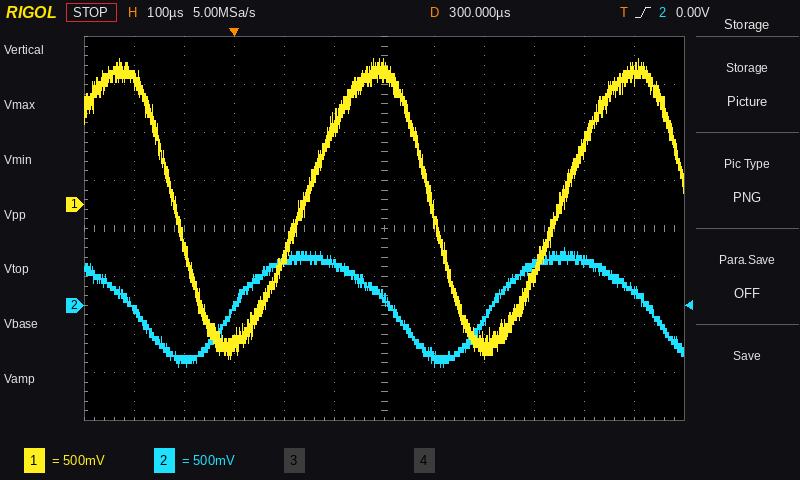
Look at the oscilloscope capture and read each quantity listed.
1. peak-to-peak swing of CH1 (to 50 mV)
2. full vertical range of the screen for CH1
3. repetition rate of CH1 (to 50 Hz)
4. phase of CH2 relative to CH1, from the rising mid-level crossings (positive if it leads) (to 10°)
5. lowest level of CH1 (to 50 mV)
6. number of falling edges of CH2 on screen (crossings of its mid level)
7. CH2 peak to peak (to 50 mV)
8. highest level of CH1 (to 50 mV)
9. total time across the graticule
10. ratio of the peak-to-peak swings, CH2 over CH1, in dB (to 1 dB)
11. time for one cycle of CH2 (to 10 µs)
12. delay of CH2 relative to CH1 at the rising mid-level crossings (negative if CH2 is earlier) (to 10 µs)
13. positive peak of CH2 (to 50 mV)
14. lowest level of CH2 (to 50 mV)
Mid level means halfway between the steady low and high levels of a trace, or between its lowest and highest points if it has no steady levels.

3.10 V
4 V
1.95 kHz
+100°
-1.60 V
3
1.25 V
1.50 V
1.2 ms
-8 dB
520 µs
-140 µs
600 mV
-650 mV
